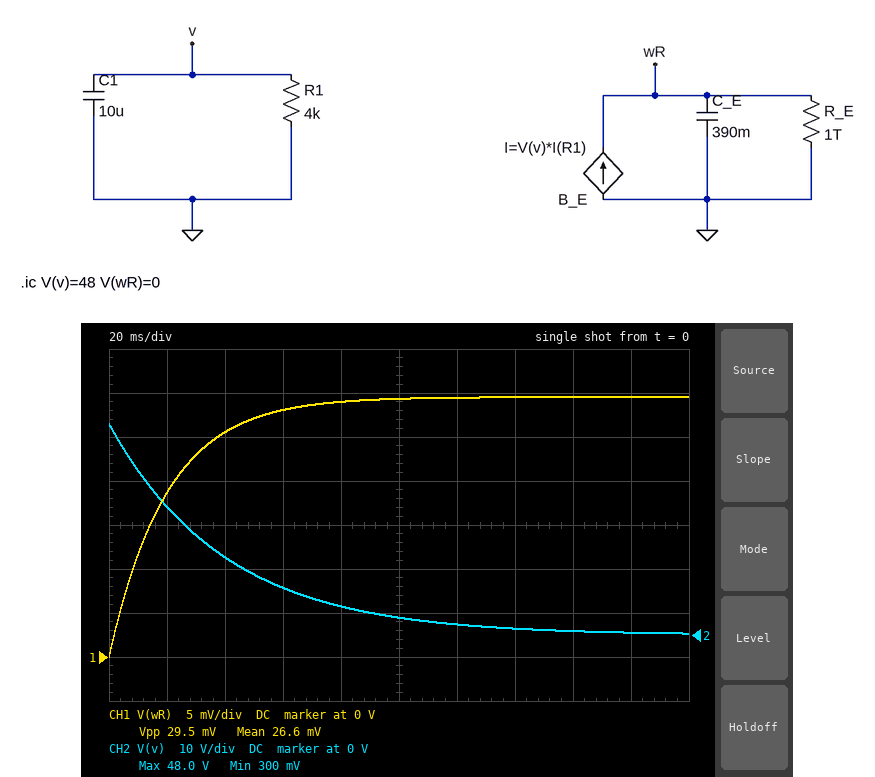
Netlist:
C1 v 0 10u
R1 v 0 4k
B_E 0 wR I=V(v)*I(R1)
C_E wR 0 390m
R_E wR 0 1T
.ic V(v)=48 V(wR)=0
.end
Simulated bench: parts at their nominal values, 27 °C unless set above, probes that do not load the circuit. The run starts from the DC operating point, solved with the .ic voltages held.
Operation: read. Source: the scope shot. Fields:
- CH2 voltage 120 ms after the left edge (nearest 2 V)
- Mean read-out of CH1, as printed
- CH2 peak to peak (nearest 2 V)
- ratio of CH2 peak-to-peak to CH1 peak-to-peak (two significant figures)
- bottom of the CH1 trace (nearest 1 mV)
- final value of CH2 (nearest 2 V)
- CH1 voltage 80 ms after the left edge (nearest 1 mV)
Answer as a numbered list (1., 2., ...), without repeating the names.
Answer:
1. 2 V
2. 26.6 mV
3. 48 V
4. 1600
5. 0 V
6. 0 V
7. 29 mV
